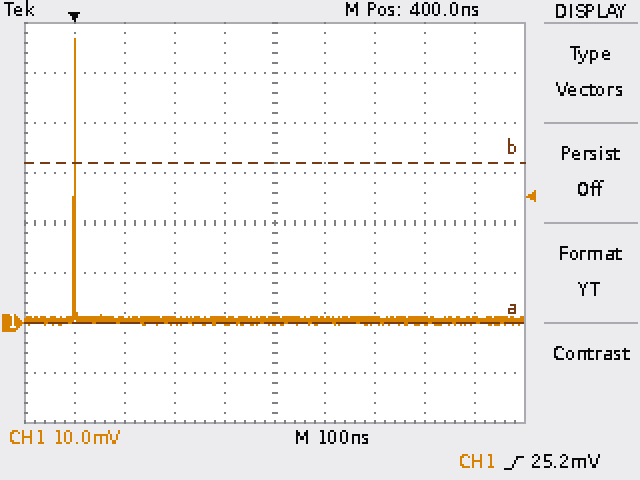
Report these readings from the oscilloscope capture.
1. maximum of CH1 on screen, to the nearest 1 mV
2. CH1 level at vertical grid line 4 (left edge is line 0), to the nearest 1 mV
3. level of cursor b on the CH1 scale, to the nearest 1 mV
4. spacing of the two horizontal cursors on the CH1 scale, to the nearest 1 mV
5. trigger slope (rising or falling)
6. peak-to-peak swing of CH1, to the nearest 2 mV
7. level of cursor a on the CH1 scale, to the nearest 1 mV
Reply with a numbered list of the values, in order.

1. 57 mV
2. 0 mV
3. 32 mV
4. 32 mV
5. rising
6. 58 mV
7. 0 mV
